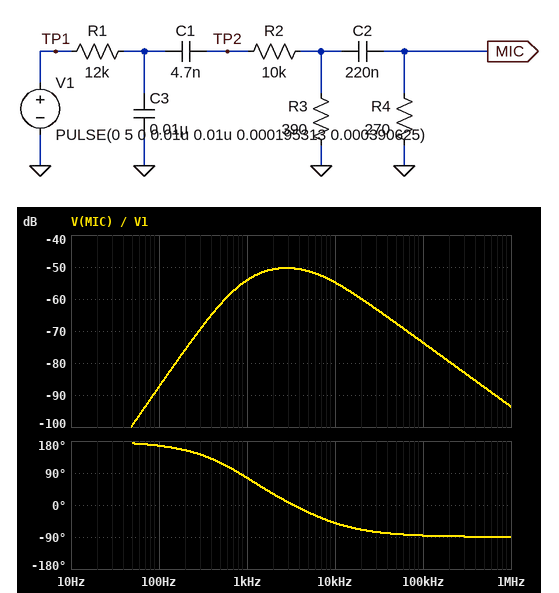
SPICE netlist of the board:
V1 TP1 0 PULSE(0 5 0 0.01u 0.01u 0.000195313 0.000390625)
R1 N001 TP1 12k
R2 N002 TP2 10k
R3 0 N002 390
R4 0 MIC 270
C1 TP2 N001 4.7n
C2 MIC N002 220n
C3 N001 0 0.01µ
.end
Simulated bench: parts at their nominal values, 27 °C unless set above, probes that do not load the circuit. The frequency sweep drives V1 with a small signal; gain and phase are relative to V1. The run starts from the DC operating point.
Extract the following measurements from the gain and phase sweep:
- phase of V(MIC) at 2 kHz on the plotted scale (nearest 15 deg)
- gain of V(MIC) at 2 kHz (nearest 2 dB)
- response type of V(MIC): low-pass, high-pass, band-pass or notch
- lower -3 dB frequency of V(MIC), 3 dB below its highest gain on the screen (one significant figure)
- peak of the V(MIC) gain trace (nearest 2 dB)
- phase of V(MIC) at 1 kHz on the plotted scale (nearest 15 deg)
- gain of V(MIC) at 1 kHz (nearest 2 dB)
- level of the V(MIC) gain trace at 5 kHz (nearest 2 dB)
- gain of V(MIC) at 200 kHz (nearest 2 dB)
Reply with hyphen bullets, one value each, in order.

- 30 deg
- -50 dB
- band-pass
- 1 kHz
- -50 dB
- 75 deg
- -54 dB
- -52 dB
- -80 dB
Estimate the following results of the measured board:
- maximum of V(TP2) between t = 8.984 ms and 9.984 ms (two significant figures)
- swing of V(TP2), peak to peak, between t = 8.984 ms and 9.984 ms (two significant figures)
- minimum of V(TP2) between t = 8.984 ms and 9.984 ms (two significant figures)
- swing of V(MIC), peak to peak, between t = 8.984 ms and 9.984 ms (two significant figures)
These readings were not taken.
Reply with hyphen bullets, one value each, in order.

- 600 mV
- 1.2 V
- -600 mV
- 21 mV
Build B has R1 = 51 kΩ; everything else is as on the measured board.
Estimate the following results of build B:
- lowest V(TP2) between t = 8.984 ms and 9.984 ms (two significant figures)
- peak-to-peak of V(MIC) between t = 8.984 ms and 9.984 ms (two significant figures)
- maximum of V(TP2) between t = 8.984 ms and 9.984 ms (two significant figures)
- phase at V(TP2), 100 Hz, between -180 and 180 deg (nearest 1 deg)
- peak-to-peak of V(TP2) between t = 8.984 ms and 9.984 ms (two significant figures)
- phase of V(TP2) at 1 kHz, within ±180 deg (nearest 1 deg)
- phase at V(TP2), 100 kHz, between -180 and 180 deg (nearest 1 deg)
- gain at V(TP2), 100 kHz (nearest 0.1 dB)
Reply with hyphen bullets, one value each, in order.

- -150 mV
- 4.9 mV
- 150 mV
- 63 deg
- 300 mV
- 0 deg
- -87 deg
- -50.1 dB
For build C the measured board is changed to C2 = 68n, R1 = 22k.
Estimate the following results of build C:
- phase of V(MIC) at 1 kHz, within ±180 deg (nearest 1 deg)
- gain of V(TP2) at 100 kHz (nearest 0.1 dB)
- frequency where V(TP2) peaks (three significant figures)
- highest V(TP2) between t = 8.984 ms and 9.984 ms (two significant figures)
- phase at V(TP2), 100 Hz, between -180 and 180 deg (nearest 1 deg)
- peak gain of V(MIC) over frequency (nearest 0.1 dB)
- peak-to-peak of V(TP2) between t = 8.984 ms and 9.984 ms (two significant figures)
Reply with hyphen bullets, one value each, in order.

- 88 deg
- -42.8 dB
- 1.50 kHz
- 340 mV
- 77 deg
- -57.8 dB
- 680 mV
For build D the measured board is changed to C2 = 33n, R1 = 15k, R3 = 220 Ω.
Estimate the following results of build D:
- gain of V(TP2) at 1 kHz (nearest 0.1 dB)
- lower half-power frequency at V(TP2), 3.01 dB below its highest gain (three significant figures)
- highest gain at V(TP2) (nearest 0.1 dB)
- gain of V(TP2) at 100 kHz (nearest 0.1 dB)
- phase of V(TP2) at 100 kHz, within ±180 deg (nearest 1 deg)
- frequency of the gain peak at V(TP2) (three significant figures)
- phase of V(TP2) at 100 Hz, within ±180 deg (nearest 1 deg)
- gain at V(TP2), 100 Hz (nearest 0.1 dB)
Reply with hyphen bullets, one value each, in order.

- -15.7 dB
- 542 Hz
- -15.0 dB
- -39.5 dB
- -87 deg
- 1.87 kHz
- 80 deg
- -30.5 dB
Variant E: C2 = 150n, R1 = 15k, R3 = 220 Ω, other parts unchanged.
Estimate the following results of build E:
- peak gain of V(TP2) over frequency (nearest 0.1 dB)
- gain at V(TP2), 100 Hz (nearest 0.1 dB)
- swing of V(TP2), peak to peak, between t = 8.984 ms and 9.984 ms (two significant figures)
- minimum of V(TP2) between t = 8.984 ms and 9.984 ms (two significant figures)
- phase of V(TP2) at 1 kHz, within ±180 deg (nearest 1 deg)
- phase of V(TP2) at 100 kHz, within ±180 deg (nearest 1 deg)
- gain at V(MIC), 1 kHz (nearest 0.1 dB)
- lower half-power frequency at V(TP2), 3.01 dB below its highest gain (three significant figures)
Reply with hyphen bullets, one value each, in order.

- -15.0 dB
- -30.5 dB
- 980 mV
- -490 mV
- 23 deg
- -87 deg
- -61.7 dB
- 539 Hz
